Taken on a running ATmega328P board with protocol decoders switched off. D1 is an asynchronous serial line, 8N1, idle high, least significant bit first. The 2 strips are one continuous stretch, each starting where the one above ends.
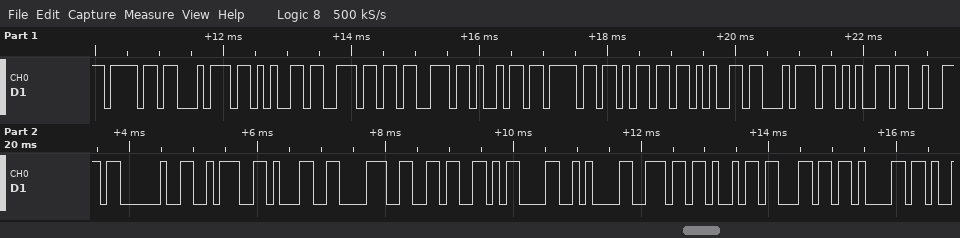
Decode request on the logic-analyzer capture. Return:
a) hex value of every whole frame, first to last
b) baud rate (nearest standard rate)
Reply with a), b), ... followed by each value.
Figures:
a) 6F 74 65 6E 73 69 6F 6D 65 74 65 72 20 3A 31 38 36 0D 0A 6E 69 6C 61
b) 9600 baud
